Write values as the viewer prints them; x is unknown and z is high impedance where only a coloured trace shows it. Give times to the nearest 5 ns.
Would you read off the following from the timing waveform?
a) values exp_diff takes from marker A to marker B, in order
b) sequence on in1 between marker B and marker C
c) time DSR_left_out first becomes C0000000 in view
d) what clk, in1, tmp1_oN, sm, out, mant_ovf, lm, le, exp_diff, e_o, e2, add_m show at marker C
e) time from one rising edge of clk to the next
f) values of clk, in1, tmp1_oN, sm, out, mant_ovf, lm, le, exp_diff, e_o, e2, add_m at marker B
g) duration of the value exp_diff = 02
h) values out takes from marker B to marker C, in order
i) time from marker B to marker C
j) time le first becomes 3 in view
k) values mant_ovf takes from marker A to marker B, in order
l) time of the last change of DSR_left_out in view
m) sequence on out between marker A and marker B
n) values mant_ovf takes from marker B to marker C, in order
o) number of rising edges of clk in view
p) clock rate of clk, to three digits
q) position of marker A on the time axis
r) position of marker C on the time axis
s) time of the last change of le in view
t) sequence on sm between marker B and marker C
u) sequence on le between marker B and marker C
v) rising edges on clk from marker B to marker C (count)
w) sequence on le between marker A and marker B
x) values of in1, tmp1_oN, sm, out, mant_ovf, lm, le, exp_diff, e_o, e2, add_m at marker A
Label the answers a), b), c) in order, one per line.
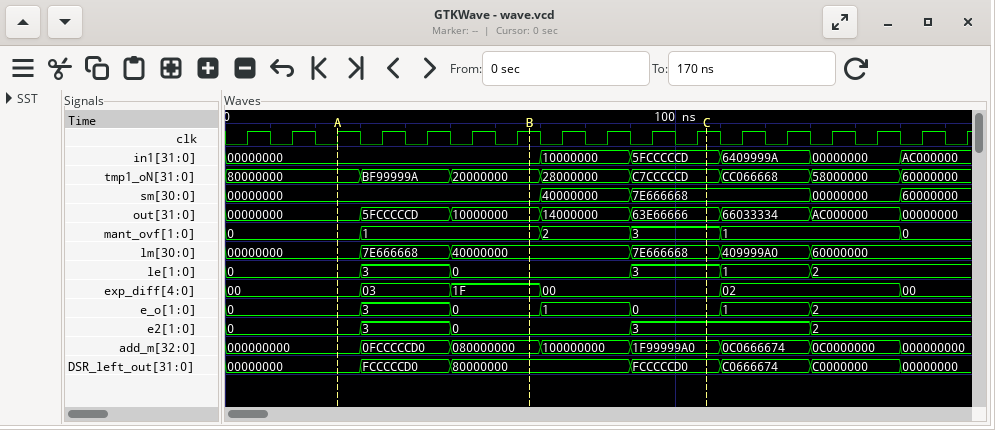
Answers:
a) 00, 03, 1F
b) 00000000, 10000000, 5FCCCCCD
c) 130 ns
d) clk=1, in1=5FCCCCCD, tmp1_oN=C7CCCCCD, sm=7E666668, out=63E66666, mant_ovf=3, lm=7E666668, le=3, exp_diff=00, e_o=0, e2=3, add_m=1F99999A0
e) 10 ns
f) clk=1, in1=00000000, tmp1_oN=20000000, sm=00000000, out=10000000, mant_ovf=1, lm=40000000, le=0, exp_diff=1F, e_o=0, e2=0, add_m=080000000
g) 40 ns
h) 10000000, 14000000, 63E66666
i) 40 ns
j) 30 ns
k) 0, 1
l) 150 ns
m) 00000000, 5FCCCCCD, 10000000
n) 1, 2, 3
o) 17
p) 100 MHz
q) 25 ns
r) 105 ns
s) 130 ns
t) 00000000, 40000000, 7E666668
u) 0, 3
v) 4
w) 0, 3, 0
x) in1=00000000, tmp1_oN=80000000, sm=00000000, out=00000000, mant_ovf=0, lm=00000000, le=0, exp_diff=00, e_o=0, e2=0, add_m=000000000
